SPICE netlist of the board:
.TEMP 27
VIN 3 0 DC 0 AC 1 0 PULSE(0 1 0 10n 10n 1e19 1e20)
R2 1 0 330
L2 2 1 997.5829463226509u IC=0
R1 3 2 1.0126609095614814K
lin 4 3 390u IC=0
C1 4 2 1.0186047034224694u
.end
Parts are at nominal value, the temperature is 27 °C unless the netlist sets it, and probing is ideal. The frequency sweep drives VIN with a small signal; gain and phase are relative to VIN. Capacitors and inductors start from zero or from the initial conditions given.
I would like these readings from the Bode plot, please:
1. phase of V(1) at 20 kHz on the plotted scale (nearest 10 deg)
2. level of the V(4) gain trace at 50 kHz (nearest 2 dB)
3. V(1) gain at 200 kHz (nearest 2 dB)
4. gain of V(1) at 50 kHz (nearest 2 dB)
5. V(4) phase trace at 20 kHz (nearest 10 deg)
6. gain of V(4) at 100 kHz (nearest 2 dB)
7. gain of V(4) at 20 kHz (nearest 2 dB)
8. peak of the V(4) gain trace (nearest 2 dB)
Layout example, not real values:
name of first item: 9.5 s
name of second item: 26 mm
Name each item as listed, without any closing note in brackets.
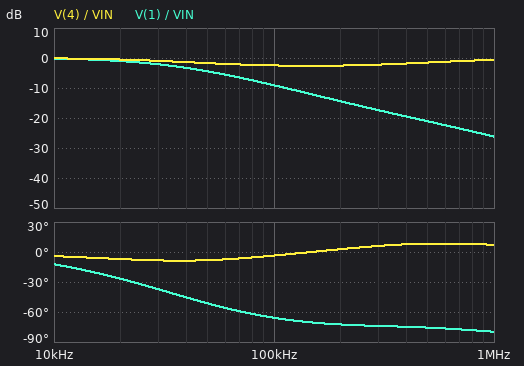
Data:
phase of V(1) at 20 kHz on the plotted scale: -30 deg
level of the V(4) gain trace at 50 kHz: -2 dB
V(1) gain at 200 kHz: -14 dB
gain of V(1) at 50 kHz: -4 dB
V(4) phase trace at 20 kHz: -10 deg
gain of V(4) at 100 kHz: -2 dB
gain of V(4) at 20 kHz: 0 dB
peak of the V(4) gain trace: 0 dB
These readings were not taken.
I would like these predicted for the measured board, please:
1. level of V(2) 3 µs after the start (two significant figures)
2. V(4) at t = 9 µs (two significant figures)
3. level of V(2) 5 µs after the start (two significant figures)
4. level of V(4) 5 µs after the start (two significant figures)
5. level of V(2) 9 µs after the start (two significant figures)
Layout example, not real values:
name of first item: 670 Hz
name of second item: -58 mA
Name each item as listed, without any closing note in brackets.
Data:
level of V(2) 3 µs after the start: 850 mV
V(4) at t = 9 µs: 970 mV
level of V(2) 5 µs after the start: 900 mV
level of V(4) 5 µs after the start: 910 mV
level of V(2) 9 µs after the start: 950 mV
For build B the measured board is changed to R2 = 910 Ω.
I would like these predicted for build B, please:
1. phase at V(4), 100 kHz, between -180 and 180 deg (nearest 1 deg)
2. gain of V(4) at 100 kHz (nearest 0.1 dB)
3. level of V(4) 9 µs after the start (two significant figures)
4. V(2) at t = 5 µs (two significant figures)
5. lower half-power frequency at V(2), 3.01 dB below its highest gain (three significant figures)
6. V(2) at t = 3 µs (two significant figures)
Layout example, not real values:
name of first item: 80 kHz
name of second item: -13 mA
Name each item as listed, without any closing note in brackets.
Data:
phase at V(4), 100 kHz, between -180 and 180 deg: -7 deg
gain of V(4) at 100 kHz: -1.4 dB
level of V(4) 9 µs after the start: 1.0 V
V(2) at t = 5 µs: 980 mV
lower half-power frequency at V(2), 3.01 dB below its highest gain: 242 Hz
V(2) at t = 3 µs: 950 mV
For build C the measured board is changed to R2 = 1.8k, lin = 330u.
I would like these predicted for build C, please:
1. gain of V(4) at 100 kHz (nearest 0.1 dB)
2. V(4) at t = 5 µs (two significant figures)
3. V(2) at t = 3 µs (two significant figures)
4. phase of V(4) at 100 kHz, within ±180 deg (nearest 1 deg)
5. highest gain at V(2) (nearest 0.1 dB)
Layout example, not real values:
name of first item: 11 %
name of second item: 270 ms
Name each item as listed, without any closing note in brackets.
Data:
gain of V(4) at 100 kHz: -0.5 dB
V(4) at t = 5 µs: 1.0 V
V(2) at t = 3 µs: 990 mV
phase of V(4) at 100 kHz, within ±180 deg: -5 deg
highest gain at V(2): 0 dB
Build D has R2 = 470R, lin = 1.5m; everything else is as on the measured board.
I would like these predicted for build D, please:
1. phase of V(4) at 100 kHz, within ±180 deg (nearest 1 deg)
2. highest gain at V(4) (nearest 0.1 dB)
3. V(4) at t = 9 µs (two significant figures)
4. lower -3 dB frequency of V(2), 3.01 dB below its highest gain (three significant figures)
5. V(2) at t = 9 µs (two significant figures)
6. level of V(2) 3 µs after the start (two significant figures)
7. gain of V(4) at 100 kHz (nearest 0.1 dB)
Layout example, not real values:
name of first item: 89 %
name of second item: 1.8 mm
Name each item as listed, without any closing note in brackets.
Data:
phase of V(4) at 100 kHz, within ±180 deg: 3 deg
highest gain at V(4): 0.1 dB
V(4) at t = 9 µs: 870 mV
lower -3 dB frequency of V(2), 3.01 dB below its highest gain: 429 Hz
V(2) at t = 9 µs: 860 mV
level of V(2) 3 µs after the start: 660 mV
gain of V(4) at 100 kHz: -5.5 dB
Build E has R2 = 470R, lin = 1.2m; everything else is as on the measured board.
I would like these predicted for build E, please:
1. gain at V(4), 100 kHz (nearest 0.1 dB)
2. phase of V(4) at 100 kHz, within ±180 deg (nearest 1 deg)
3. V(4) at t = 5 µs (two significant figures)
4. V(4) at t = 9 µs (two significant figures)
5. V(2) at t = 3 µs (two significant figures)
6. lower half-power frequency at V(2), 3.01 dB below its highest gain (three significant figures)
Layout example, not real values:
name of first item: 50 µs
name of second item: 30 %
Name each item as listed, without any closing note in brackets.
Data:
gain at V(4), 100 kHz: -5.0 dB
phase of V(4) at 100 kHz, within ±180 deg: 0 deg
V(4) at t = 5 µs: 800 mV
V(4) at t = 9 µs: 910 mV
V(2) at t = 3 µs: 700 mV
lower half-power frequency at V(2), 3.01 dB below its highest gain: 430 Hz
